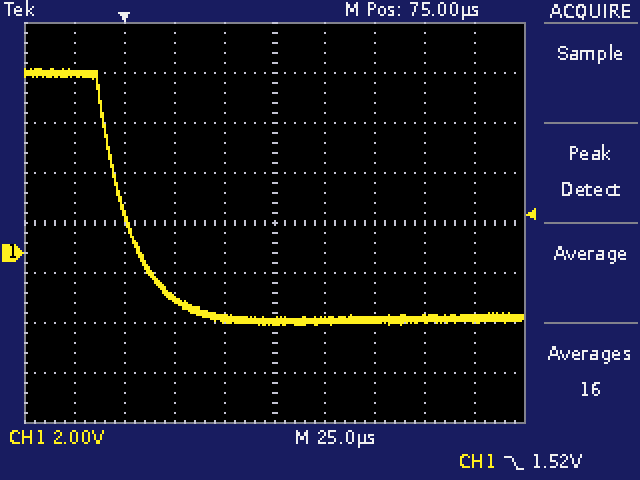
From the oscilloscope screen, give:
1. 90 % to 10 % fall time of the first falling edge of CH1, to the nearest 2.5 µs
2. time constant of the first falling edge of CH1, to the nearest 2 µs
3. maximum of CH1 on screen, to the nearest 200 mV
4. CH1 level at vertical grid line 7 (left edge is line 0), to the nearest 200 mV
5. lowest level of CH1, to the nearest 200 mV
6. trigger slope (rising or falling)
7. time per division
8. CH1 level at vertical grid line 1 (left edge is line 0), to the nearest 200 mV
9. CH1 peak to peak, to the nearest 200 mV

35.0 µs
16 µs
7.4 V
-2.6 V
-2.8 V
falling
25 µs
7.2 V
10.2 V
